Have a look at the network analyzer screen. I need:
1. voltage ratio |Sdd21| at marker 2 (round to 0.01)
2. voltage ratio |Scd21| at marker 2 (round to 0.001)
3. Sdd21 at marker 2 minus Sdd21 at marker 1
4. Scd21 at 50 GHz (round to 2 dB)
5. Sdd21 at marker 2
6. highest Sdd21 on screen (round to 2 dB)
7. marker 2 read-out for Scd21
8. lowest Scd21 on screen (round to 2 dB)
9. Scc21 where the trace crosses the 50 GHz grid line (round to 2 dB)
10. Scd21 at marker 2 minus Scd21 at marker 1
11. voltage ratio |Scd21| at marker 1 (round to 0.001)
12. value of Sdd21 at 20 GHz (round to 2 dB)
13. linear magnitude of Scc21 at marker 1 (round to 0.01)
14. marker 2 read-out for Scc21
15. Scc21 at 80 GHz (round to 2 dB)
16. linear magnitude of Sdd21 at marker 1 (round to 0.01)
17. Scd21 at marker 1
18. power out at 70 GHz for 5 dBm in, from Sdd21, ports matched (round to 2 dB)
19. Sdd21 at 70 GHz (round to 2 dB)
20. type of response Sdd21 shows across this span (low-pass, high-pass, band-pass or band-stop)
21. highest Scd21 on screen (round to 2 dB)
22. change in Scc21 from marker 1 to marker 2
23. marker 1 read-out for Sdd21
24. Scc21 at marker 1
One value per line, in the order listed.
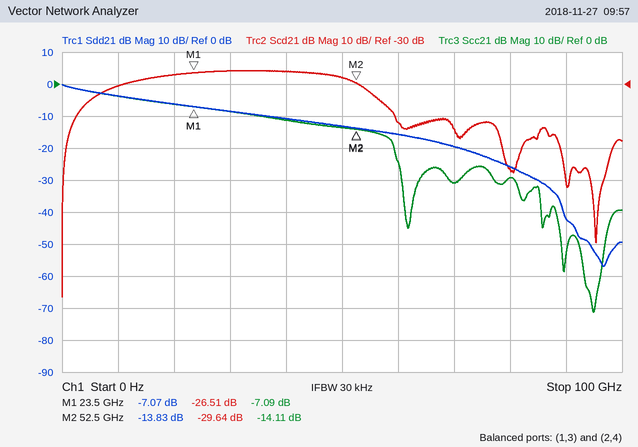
0.20
0.033
-6.76 dB
-28 dB
-13.83 dB
0 dB
-29.64 dB
-96 dB
-14 dB
-3.13 dB
0.047
-6 dB
0.44
-14.11 dB
-30 dB
0.44
-26.51 dB
-14 dBm
-20 dB
low-pass
-26 dB
-7.02 dB
-7.07 dB
-7.09 dB
